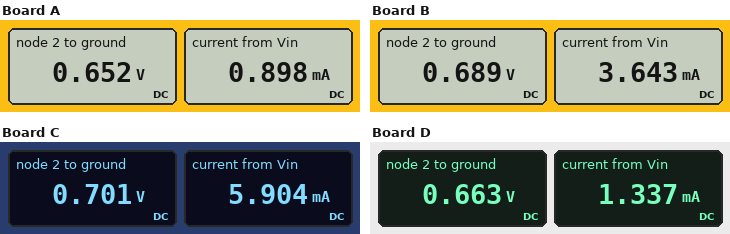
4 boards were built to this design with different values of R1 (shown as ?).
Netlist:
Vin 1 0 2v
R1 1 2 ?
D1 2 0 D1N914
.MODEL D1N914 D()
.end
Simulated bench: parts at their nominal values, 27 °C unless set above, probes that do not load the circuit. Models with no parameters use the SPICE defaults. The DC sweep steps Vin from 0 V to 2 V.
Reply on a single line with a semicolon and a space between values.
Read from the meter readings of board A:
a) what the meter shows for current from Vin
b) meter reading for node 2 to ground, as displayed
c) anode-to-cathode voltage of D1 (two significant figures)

0.898 mA; 0.652 V; 650 mV
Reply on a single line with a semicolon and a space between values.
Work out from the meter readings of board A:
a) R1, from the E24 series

1.5 kΩ
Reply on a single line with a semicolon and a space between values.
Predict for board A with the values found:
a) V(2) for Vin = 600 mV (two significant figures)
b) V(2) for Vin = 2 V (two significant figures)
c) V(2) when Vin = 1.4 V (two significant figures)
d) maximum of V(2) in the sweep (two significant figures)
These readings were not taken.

560 mV; 650 mV; 640 mV; 650 mV
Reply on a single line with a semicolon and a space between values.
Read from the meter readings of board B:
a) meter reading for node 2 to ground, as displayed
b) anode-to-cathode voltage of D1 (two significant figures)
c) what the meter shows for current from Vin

0.689 V; 690 mV; 3.643 mA
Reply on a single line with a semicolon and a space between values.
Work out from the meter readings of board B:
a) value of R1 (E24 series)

360 Ω
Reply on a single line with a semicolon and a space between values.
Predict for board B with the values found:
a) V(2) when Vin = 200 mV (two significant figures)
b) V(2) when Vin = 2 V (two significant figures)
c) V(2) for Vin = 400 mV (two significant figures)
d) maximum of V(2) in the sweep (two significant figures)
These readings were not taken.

200 mV; 690 mV; 400 mV; 690 mV
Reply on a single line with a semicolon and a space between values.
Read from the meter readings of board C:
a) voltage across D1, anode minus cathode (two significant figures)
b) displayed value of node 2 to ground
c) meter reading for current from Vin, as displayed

700 mV; 0.701 V; 5.904 mA
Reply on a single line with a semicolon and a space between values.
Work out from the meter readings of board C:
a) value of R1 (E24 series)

220 Ω
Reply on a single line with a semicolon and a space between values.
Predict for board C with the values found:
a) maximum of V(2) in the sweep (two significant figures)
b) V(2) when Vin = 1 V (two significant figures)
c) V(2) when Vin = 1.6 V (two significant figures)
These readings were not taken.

700 mV; 670 mV; 690 mV
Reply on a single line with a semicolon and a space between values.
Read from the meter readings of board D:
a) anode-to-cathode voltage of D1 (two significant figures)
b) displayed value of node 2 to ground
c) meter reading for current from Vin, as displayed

660 mV; 0.663 V; 1.337 mA
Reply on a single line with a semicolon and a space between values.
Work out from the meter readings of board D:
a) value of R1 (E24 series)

1 kΩ
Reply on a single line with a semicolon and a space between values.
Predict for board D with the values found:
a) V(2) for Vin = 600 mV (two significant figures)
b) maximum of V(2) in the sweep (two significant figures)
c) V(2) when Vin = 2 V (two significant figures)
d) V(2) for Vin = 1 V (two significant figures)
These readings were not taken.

570 mV; 660 mV; 660 mV; 630 mV
